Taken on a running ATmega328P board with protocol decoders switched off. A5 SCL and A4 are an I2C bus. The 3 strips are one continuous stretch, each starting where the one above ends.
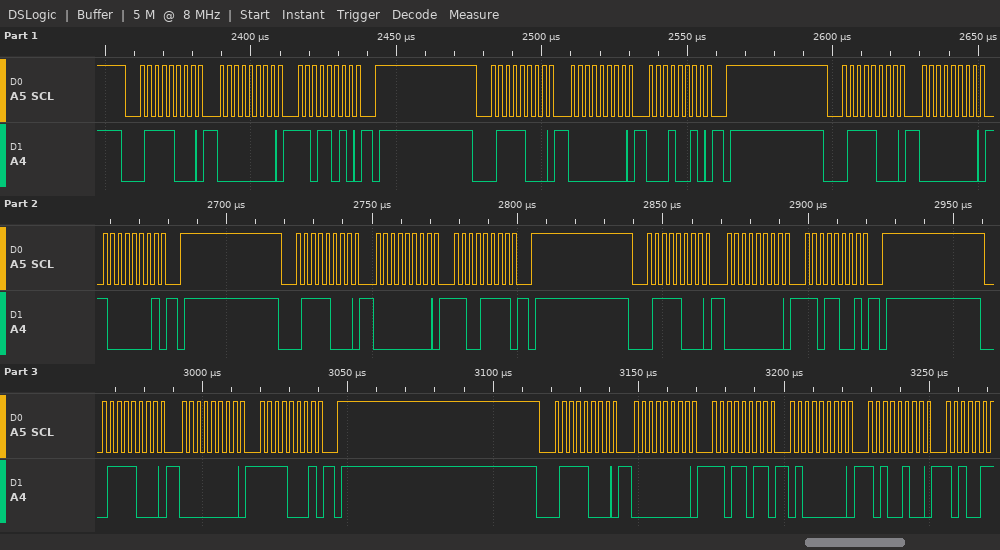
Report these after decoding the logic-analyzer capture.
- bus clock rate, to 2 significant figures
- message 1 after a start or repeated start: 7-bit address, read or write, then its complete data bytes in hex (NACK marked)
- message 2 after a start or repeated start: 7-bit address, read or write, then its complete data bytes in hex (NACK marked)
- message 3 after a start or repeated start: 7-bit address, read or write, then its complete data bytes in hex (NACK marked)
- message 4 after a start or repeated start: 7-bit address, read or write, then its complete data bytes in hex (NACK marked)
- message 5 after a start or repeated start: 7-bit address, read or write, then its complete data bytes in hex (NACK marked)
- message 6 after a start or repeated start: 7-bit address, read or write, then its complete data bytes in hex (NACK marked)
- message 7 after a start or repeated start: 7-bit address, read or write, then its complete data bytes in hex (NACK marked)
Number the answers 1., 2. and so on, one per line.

1. 400 kHz
2. 0x3C write: 00 DA
3. 0x3C write: 00 12
4. 0x3C write: 00 81
5. 0x3C write: 00 CF
6. 0x3C write: 00 D9
7. 0x3C write: 00 F1
8. 0x3C write: 00 DB 40 A4
